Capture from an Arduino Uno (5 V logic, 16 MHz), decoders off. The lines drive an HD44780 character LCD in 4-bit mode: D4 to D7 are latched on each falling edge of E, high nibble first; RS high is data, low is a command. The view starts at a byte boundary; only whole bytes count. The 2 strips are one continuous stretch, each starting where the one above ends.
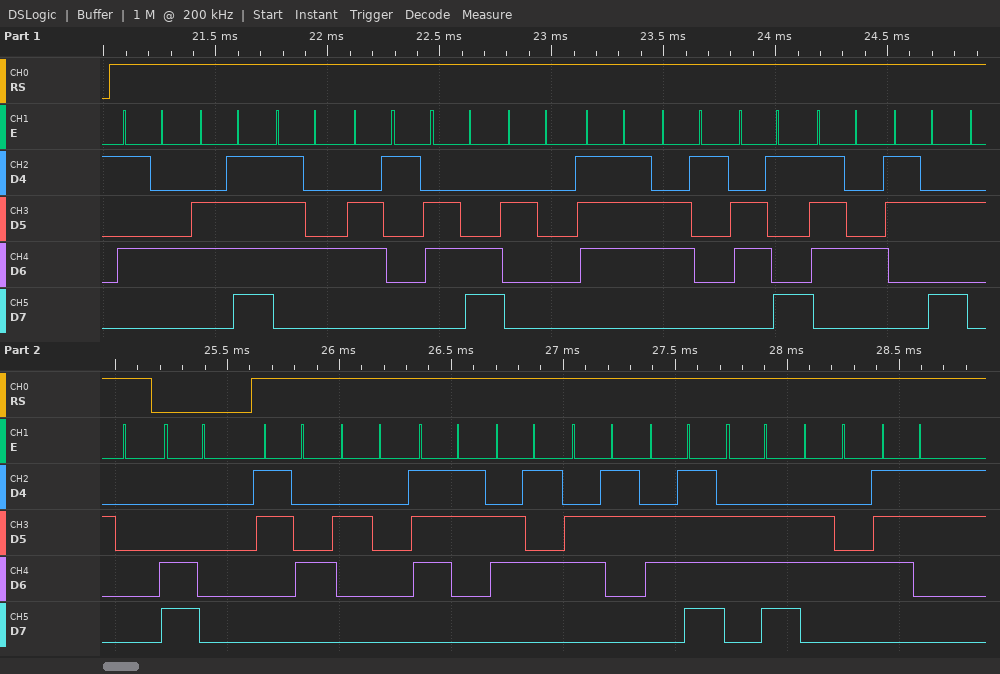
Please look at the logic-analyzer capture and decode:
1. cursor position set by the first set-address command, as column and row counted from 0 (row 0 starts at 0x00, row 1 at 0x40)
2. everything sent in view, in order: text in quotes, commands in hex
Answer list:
column 0, row 1
"Total wait: " 0xC0 "4 seconds"
